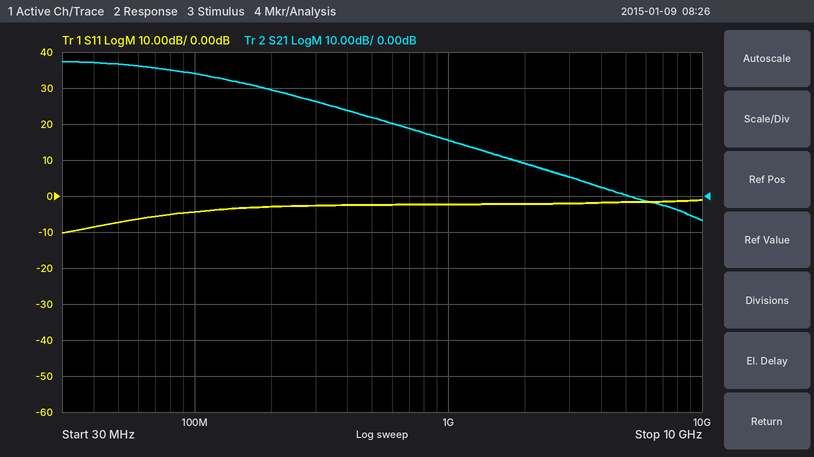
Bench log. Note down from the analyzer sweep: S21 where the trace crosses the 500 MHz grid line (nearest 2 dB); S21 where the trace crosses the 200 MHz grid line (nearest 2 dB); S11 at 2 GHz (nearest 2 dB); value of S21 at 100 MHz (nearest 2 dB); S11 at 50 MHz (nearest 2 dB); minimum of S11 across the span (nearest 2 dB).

22 dB
30 dB
-2 dB
34 dB
-8 dB
-10 dB
